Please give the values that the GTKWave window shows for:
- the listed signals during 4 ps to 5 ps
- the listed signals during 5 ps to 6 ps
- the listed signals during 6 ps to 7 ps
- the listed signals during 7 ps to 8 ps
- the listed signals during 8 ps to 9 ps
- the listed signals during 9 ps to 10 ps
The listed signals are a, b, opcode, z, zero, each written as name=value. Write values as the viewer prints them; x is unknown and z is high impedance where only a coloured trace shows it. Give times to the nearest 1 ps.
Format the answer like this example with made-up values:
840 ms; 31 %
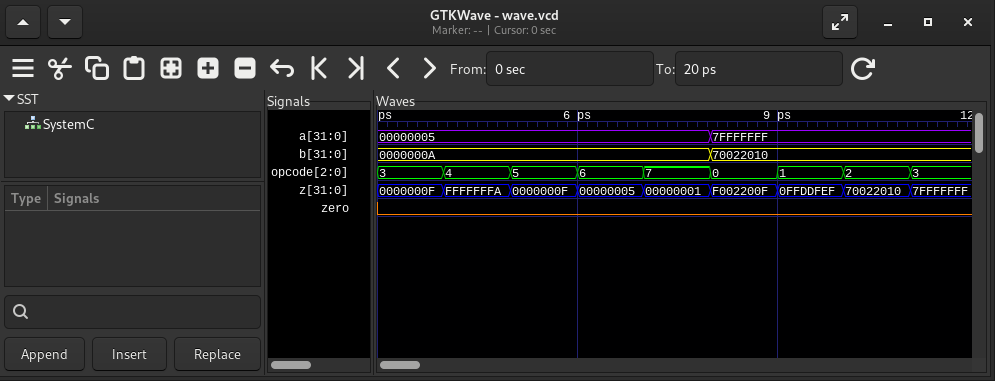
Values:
a=00000005, b=0000000A, opcode=4, z=FFFFFFFA, zero=0; a=00000005, b=0000000A, opcode=5, z=0000000F, zero=0; a=00000005, b=0000000A, opcode=6, z=00000005, zero=0; a=00000005, b=0000000A, opcode=7, z=00000001, zero=0; a=7FFFFFFF, b=70022010, opcode=0, z=F002200F, zero=0; a=7FFFFFFF, b=70022010, opcode=1, z=0FFDDFEF, zero=0
